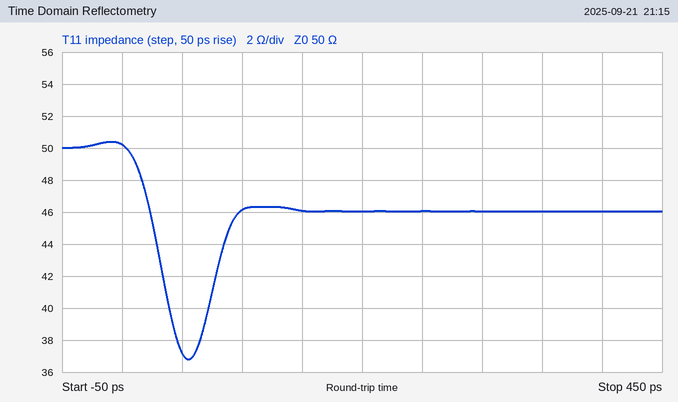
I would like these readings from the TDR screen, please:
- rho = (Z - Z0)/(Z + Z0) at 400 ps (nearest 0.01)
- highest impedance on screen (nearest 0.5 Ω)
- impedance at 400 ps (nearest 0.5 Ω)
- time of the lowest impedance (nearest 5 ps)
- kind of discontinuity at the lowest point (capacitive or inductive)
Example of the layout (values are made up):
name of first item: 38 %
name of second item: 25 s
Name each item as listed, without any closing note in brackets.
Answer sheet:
rho = (Z - Z0)/(Z + Z0) at 400 ps: -0.04
highest impedance on screen: 50.5 Ω
impedance at 400 ps: 46.0 Ω
time of the lowest impedance: 55 ps
kind of discontinuity at the lowest point: capacitive
